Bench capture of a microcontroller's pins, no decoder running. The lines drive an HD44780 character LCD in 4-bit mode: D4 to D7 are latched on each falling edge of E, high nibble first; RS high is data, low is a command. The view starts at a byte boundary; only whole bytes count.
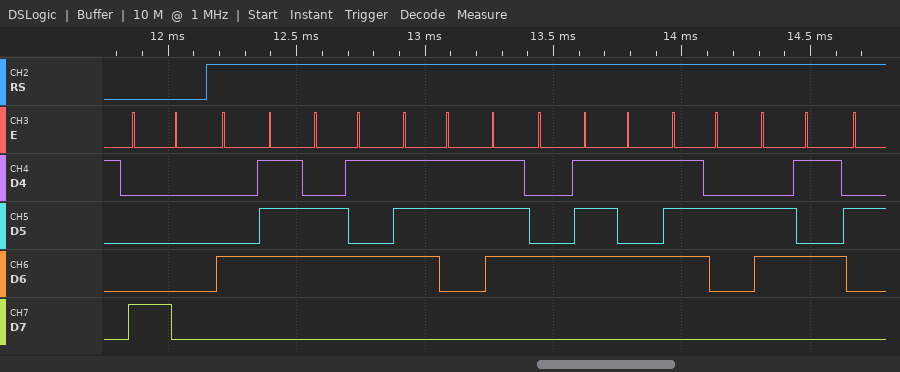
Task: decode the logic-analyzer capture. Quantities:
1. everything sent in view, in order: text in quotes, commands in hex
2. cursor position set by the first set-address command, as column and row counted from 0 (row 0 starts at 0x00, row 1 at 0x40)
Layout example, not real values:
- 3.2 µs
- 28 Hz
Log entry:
- 0x80 "Gesture"
- column 0, row 0
